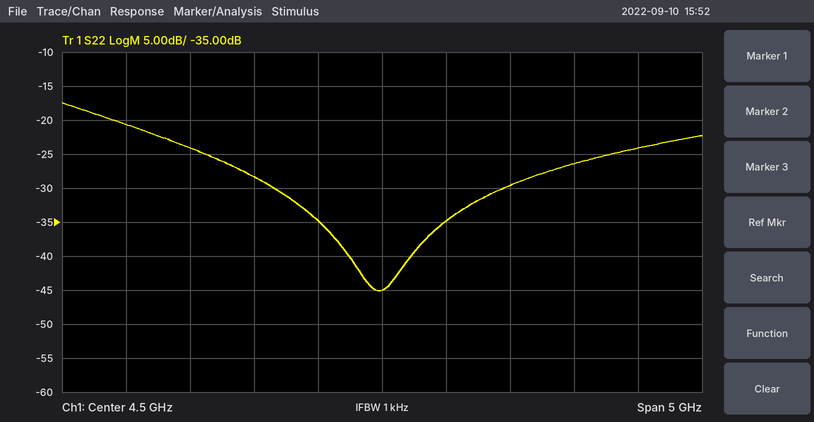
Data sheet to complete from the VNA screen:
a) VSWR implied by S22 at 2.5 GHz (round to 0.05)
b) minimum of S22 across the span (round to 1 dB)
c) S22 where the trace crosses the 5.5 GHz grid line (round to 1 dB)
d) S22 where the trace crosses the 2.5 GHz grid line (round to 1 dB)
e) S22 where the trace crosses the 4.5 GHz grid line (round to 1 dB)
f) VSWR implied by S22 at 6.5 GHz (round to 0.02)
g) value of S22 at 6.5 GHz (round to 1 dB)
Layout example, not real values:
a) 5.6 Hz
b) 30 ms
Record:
a) 1.20
b) -45 dB
c) -30 dB
d) -21 dB
e) -45 dB
f) 1.14
g) -24 dB
